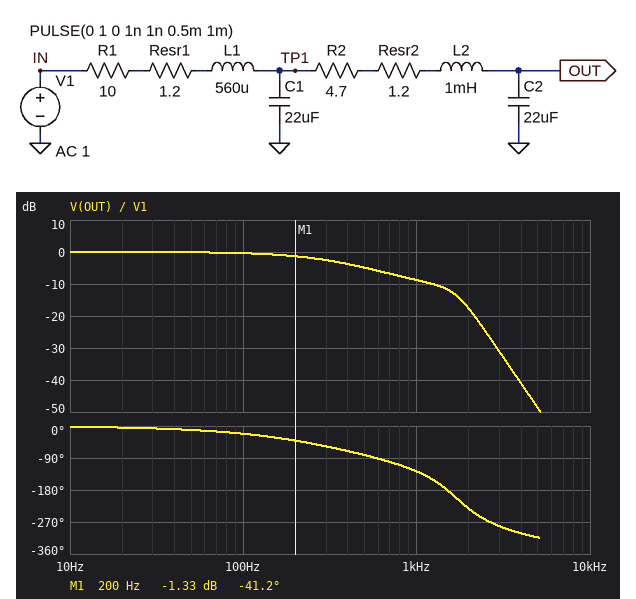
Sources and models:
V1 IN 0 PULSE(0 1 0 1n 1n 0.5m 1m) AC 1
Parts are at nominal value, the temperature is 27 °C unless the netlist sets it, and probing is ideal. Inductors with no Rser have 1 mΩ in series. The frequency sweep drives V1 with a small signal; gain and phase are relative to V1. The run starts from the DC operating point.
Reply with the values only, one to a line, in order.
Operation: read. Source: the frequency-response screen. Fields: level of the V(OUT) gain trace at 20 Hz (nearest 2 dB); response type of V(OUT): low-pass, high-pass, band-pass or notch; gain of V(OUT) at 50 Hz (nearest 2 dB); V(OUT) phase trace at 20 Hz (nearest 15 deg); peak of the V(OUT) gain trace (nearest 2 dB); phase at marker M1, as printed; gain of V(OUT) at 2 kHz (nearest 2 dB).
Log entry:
0 dB
low-pass
0 dB
0 deg
0 dB
-41.2 deg
-18 dB
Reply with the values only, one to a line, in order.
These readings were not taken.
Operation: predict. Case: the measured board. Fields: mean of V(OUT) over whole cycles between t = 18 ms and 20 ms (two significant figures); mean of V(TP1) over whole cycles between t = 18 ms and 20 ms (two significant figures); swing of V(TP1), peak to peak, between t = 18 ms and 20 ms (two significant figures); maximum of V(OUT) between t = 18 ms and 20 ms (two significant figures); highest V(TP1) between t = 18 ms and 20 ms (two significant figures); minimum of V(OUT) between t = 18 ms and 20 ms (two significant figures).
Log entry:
500 mV
500 mV
370 mV
730 mV
690 mV
270 mV
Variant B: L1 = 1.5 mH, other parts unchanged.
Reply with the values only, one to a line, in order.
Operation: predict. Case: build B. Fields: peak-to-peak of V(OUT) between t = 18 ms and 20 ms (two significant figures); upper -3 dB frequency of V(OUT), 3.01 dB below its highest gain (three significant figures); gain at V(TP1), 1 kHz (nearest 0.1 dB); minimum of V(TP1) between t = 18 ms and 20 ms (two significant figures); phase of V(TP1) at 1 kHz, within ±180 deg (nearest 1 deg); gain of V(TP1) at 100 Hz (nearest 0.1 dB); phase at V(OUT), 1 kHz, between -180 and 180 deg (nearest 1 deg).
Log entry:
430 mV
389 Hz
-11.2 dB
320 mV
-69 deg
-0.3 dB
-150 deg
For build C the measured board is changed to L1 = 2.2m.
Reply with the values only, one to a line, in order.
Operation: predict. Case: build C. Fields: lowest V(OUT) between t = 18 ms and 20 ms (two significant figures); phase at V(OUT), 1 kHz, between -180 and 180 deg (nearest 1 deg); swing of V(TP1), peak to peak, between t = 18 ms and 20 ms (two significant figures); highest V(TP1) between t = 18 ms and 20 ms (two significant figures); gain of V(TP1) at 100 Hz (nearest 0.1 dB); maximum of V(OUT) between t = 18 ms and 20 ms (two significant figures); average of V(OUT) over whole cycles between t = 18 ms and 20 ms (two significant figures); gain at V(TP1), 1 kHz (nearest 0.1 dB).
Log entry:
310 mV
-163 deg
320 mV
660 mV
-0.2 dB
690 mV
500 mV
-12.4 dB
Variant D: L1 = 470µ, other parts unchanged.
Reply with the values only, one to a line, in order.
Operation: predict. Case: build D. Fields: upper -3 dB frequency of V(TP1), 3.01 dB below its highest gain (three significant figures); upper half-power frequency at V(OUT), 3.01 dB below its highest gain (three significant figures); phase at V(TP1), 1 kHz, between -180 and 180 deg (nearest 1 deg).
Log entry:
300 Hz
333 Hz
-45 deg
